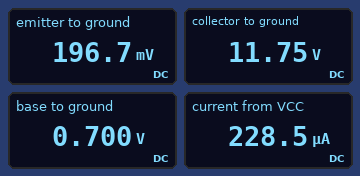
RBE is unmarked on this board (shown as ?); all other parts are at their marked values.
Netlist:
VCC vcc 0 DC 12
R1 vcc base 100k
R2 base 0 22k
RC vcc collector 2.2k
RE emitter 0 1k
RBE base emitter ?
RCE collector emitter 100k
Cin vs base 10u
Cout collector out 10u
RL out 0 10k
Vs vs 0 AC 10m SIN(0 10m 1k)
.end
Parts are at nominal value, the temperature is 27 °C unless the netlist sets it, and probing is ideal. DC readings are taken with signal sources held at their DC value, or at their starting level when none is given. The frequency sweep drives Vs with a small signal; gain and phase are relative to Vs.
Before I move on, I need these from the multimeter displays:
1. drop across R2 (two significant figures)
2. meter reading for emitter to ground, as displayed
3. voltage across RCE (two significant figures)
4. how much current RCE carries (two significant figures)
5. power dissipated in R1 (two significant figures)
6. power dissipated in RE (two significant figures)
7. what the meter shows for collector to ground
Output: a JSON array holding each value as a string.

["700 mV", "196.7 mV", "12 V", "120 µA", "1.3 mW", "39 µW", "11.75 V"]
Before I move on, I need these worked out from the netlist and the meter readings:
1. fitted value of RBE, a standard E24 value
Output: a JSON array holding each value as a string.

["6.2 kΩ"]
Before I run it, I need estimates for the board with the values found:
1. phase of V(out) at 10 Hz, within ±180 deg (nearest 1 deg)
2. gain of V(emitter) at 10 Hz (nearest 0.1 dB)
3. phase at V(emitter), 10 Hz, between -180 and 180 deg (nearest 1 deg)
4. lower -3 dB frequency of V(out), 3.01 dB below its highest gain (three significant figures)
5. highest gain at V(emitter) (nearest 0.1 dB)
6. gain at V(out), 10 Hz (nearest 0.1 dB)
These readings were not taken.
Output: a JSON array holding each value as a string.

["25 deg", "-17.6 dB", "17 deg", "3.55 Hz", "-17.2 dB", "-52.7 dB"]
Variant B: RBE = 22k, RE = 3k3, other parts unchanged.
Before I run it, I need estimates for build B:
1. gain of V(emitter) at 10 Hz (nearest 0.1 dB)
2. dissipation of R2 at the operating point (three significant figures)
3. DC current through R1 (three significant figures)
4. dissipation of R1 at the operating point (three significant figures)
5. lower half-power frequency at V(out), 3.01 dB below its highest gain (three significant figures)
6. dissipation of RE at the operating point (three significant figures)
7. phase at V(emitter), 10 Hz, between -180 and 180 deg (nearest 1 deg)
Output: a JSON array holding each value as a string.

["-18.0 dB", "91.4 µW", "106 µA", "1.12 mW", "2.20 Hz", "78.1 µW", "9 deg"]
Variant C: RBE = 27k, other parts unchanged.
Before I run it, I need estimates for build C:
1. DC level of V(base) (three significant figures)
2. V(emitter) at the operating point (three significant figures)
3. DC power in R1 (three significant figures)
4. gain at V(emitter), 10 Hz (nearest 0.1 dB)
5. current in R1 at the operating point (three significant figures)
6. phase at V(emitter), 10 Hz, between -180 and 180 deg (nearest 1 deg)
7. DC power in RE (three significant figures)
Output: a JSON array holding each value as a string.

["1.36 V", "160 mV", "1.13 mW", "-29.1 dB", "106 µA", "8 deg", "25.7 µW"]
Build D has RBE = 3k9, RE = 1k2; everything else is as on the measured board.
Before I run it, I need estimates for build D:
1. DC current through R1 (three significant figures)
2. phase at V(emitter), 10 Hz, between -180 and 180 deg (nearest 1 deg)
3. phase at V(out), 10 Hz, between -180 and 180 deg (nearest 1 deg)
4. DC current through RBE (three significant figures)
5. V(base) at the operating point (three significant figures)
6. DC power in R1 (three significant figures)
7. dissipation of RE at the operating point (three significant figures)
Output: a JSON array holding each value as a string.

["114 µA", "22 deg", "29 deg", "87.6 µA", "585 mV", "1.30 mW", "49.3 µW"]
